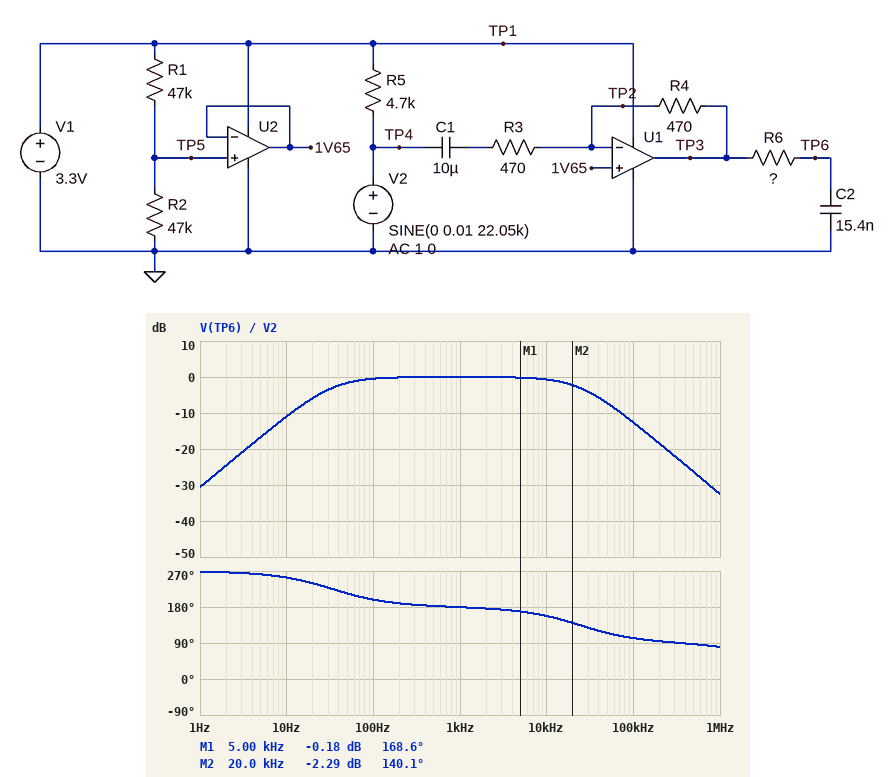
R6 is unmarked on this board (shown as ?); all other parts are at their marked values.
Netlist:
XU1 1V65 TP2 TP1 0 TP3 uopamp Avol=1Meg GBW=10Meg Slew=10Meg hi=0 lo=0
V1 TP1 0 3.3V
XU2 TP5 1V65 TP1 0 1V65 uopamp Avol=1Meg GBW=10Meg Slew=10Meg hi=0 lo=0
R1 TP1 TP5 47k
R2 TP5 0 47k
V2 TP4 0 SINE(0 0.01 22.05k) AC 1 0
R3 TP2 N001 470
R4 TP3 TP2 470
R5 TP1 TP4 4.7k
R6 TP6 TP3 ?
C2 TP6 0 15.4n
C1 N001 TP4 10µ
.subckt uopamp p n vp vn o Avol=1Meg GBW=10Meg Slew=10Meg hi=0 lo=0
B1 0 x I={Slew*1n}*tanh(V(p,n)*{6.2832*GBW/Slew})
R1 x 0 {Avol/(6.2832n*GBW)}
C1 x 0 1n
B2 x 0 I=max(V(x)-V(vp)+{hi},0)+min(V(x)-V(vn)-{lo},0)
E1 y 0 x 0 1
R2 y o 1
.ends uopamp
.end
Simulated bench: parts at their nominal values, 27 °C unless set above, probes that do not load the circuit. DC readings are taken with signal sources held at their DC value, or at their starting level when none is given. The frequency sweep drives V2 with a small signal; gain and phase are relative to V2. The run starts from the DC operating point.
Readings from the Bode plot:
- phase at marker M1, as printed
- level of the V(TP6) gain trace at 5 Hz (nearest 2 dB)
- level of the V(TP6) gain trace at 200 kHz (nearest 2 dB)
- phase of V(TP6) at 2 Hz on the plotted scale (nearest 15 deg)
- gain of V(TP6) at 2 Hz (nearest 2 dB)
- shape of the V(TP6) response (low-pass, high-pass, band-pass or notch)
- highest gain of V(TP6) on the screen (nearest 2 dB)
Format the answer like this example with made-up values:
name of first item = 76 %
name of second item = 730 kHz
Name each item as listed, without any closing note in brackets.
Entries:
phase at marker M1, as printed = 168.6 deg
level of the V(TP6) gain trace at 5 Hz = -16 dB
level of the V(TP6) gain trace at 200 kHz = -18 dB
phase of V(TP6) at 2 Hz on the plotted scale = 270 deg
gain of V(TP6) at 2 Hz = -24 dB
shape of the V(TP6) response = band-pass
highest gain of V(TP6) on the screen = 0 dB
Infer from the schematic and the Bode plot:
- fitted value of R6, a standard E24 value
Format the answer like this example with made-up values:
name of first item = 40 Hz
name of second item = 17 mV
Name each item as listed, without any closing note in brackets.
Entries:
fitted value of R6, a standard E24 value = 430 Ω
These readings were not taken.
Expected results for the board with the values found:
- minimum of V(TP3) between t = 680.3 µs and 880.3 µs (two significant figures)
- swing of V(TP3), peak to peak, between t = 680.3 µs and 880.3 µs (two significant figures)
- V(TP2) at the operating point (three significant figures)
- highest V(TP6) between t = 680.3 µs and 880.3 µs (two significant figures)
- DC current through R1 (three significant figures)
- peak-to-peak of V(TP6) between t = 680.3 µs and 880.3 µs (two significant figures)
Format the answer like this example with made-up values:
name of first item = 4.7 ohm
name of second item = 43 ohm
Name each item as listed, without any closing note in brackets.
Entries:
minimum of V(TP3) between t = 680.3 µs and 880.3 µs = 1.6 V
swing of V(TP3), peak to peak, between t = 680.3 µs and 880.3 µs = 20 mV
V(TP2) at the operating point = 1.65 V
highest V(TP6) between t = 680.3 µs and 880.3 µs = 1.7 V
DC current through R1 = 35.1 µA
peak-to-peak of V(TP6) between t = 680.3 µs and 880.3 µs = 15 mV
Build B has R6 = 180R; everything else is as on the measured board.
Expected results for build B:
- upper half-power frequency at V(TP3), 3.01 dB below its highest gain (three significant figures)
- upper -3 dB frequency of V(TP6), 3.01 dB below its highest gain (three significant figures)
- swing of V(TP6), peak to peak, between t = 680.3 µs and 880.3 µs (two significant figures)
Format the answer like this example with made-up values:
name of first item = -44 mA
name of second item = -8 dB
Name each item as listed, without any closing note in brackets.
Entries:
upper half-power frequency at V(TP3), 3.01 dB below its highest gain = 4.97 MHz
upper -3 dB frequency of V(TP6), 3.01 dB below its highest gain = 57.5 kHz
swing of V(TP6), peak to peak, between t = 680.3 µs and 880.3 µs = 19 mV
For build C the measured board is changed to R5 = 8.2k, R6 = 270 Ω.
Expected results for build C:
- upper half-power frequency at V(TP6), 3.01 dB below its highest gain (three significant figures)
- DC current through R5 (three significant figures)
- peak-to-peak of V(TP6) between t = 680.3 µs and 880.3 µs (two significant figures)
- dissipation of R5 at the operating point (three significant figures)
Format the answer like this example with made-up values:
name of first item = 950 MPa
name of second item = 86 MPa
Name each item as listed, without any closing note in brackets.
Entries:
upper half-power frequency at V(TP6), 3.01 dB below its highest gain = 38.3 kHz
DC current through R5 = 402 µA
peak-to-peak of V(TP6) between t = 680.3 µs and 880.3 µs = 17 mV
dissipation of R5 at the operating point = 1.33 mW
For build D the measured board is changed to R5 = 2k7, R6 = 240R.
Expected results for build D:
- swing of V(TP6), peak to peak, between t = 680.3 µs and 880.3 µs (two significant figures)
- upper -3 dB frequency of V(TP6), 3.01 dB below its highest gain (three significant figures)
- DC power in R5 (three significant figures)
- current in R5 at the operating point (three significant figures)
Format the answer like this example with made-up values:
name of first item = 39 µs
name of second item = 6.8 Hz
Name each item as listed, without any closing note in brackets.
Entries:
swing of V(TP6), peak to peak, between t = 680.3 µs and 880.3 µs = 18 mV
upper -3 dB frequency of V(TP6), 3.01 dB below its highest gain = 43.1 kHz
DC power in R5 = 4.03 mW
current in R5 at the operating point = 1.22 mA
